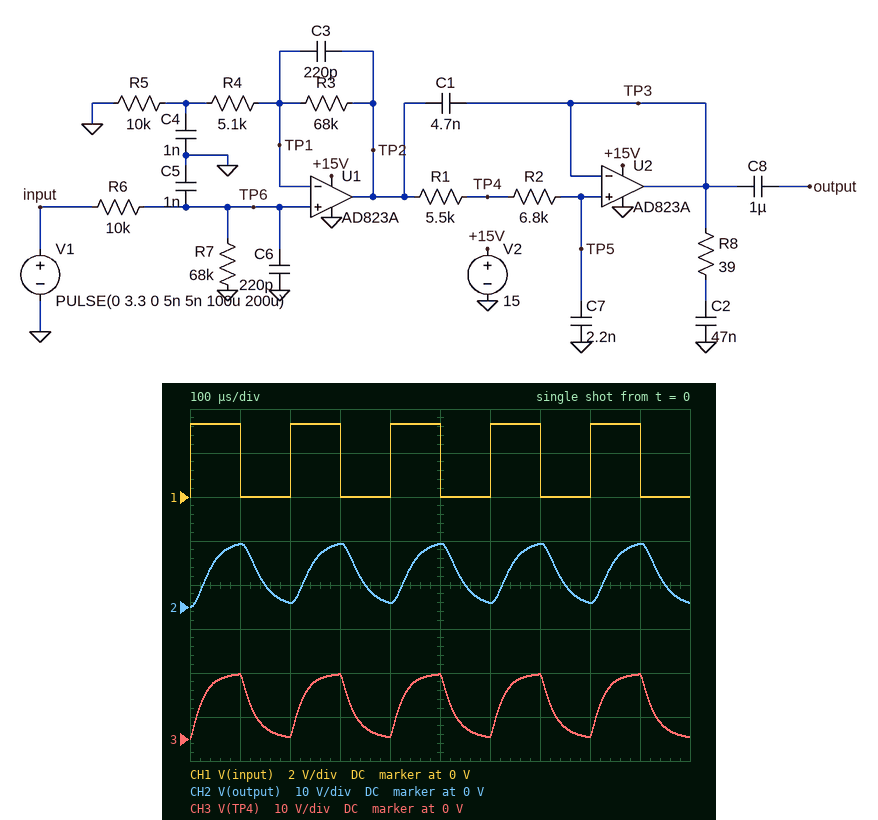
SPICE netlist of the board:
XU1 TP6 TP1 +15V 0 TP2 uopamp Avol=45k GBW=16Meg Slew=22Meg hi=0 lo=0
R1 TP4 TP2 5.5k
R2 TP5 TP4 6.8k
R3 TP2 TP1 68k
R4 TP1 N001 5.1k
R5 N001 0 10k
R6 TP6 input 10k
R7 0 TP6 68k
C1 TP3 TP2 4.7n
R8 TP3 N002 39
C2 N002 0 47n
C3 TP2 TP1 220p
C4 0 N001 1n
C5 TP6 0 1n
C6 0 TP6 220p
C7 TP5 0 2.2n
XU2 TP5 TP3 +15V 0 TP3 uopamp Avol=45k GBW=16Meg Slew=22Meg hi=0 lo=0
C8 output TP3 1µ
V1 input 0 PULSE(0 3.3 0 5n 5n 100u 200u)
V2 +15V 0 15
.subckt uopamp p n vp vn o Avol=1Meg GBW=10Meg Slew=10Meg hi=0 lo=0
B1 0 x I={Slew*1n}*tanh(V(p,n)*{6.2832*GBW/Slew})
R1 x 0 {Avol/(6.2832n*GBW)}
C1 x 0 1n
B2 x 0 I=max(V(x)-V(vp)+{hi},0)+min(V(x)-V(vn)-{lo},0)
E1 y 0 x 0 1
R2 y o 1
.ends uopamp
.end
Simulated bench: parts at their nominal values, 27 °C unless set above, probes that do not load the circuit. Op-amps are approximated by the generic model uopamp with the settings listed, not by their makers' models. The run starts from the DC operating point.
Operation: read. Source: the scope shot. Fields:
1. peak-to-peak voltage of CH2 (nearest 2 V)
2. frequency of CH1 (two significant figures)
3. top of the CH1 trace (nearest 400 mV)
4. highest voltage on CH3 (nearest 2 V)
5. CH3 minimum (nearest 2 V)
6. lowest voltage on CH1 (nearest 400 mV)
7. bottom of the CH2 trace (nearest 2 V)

14 V
5.0 kHz
3.2 V
14 V
0 V
0 V
0 V
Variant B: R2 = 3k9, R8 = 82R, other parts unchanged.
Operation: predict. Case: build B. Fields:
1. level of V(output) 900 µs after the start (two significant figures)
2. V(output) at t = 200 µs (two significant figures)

15 V
440 mV
